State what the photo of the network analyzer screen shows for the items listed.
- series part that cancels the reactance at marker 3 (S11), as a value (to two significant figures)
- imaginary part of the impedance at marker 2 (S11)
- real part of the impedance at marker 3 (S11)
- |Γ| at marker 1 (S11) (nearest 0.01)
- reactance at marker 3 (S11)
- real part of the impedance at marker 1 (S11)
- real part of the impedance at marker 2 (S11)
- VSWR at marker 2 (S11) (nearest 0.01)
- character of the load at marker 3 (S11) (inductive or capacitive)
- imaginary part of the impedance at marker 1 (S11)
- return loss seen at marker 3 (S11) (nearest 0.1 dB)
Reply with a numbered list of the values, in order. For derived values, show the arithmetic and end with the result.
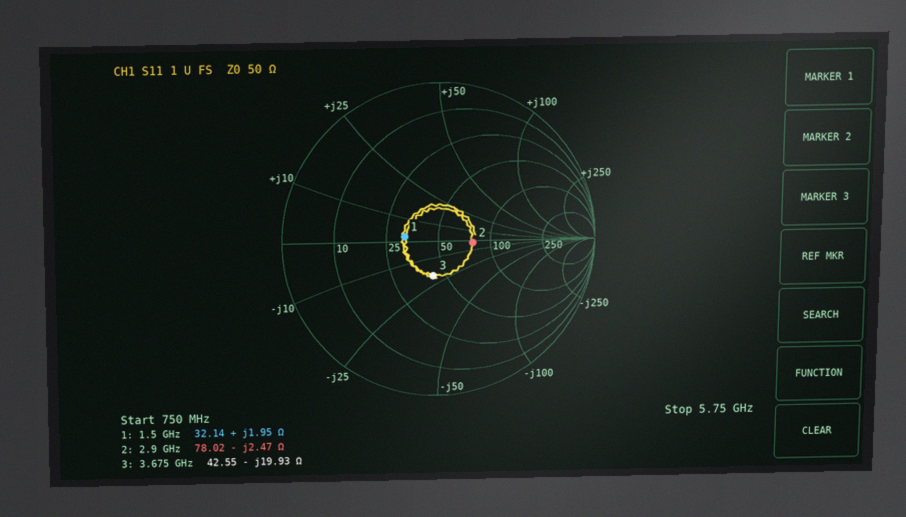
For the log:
1. L = 19.93 Ω/(2π × 3.675 GHz) ≈ 863 pH, so 860 pH to two significant figures
2. -2.47 Ω
3. 42.55 Ω
4. 0.22
5. -19.93 Ω
6. 32.14 Ω
7. 78.02 Ω
8. 1.56
9. capacitive
10. +1.95 Ω
11. 13.0 dB
